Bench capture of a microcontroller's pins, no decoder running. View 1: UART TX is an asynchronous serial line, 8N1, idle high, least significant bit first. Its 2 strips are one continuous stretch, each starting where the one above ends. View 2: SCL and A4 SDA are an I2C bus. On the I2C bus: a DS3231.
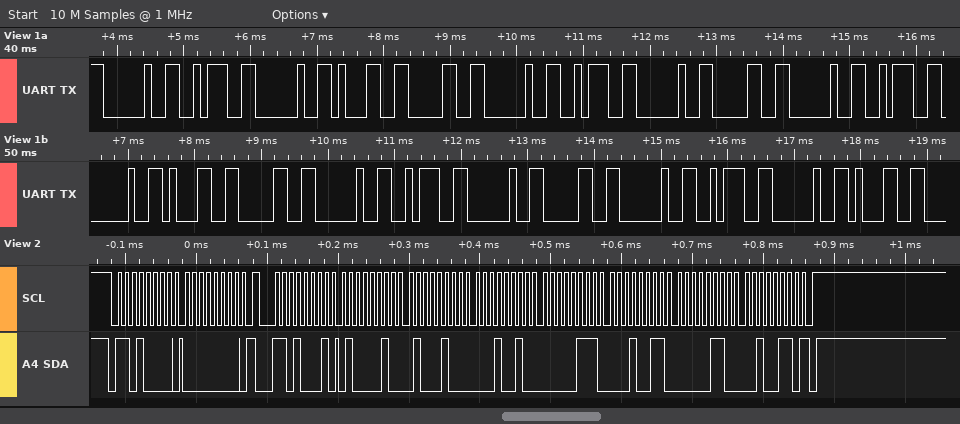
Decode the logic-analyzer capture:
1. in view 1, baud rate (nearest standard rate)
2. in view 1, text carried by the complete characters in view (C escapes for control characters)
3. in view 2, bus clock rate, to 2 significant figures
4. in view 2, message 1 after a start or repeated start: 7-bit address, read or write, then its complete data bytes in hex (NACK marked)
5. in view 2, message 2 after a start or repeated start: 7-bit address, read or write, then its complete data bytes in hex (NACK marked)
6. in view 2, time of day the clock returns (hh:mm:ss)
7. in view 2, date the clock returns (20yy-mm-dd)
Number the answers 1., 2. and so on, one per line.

1. 9600 baud
2. " : 10 : 0 : 10 : 0 : 1"
3. 100 kHz
4. 0x68 write: 00
5. 0x68 read: 42 44 12 07 13 06 26 NACK
6. 12:44:42
7. 2026-06-13
